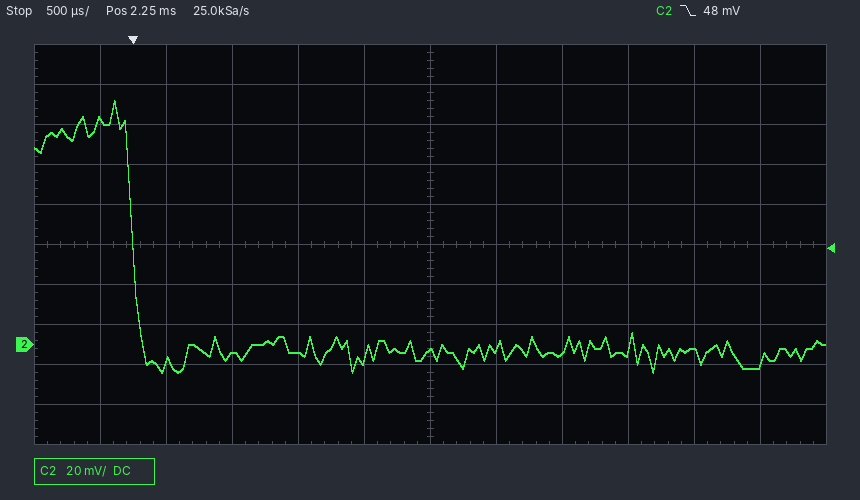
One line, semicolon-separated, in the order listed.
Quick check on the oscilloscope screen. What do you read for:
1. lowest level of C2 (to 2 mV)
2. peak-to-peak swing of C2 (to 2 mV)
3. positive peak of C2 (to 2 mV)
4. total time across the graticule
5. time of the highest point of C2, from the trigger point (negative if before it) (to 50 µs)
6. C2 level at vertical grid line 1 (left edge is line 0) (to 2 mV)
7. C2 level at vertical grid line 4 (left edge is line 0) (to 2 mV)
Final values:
-14 mV; 136 mV; 122 mV; 6 ms; -150 µs; 112 mV; -4 mV
